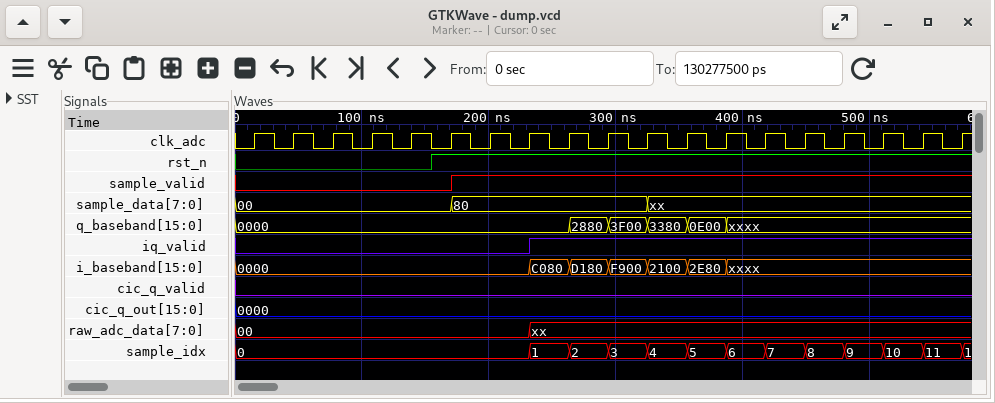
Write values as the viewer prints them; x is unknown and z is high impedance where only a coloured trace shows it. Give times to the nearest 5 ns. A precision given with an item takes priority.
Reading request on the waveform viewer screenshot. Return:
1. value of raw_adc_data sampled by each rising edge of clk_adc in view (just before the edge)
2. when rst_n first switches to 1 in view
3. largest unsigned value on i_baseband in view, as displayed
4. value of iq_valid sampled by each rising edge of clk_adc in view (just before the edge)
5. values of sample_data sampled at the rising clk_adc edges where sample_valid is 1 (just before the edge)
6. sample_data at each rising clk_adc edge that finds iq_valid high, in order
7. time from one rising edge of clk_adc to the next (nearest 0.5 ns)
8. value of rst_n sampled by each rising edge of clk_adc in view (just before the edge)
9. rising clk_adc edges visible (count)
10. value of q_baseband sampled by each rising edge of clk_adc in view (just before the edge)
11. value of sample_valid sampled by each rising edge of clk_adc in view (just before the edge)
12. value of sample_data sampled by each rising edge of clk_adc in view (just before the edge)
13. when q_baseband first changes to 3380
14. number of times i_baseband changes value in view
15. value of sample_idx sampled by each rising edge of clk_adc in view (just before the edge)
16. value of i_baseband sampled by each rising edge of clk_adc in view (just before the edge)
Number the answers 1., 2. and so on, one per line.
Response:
1. 00, 00, 00, 00, 00, 00, 00, 00, xx, xx, xx, xx, xx, xx, xx, xx, xx, xx, xx
2. 155 ns
3. F900
4. 0 0 0 0 0 0 0 0 1 1 1 1 1 1 1 1 1 1 1
5. 80, 80, 80, 80, 80, xx, xx, xx, xx, xx, xx, xx, xx
6. 80, 80, 80, xx, xx, xx, xx, xx, xx, xx, xx
7. 31 ns
8. 0 0 0 0 0 1 1 1 1 1 1 1 1 1 1 1 1 1 1
9. 19
10. 0000, 0000, 0000, 0000, 0000, 0000, 0000, 0000, 0000, 2880, 3F00, 3380, 0E00, xxxx, xxxx, xxxx, xxxx, xxxx, xxxx
11. 0 0 0 0 0 0 1 1 1 1 1 1 1 1 1 1 1 1 1
12. 00, 00, 00, 00, 00, 00, 80, 80, 80, 80, 80, xx, xx, xx, xx, xx, xx, xx, xx
13. 325 ns
14. 6
15. 0, 0, 0, 0, 0, 0, 0, 0, 1, 2, 3, 4, 5, 6, 7, 8, 9, 10, 11
16. 0000, 0000, 0000, 0000, 0000, 0000, 0000, 0000, C080, D180, F900, 2100, 2E80, xxxx, xxxx, xxxx, xxxx, xxxx, xxxx
